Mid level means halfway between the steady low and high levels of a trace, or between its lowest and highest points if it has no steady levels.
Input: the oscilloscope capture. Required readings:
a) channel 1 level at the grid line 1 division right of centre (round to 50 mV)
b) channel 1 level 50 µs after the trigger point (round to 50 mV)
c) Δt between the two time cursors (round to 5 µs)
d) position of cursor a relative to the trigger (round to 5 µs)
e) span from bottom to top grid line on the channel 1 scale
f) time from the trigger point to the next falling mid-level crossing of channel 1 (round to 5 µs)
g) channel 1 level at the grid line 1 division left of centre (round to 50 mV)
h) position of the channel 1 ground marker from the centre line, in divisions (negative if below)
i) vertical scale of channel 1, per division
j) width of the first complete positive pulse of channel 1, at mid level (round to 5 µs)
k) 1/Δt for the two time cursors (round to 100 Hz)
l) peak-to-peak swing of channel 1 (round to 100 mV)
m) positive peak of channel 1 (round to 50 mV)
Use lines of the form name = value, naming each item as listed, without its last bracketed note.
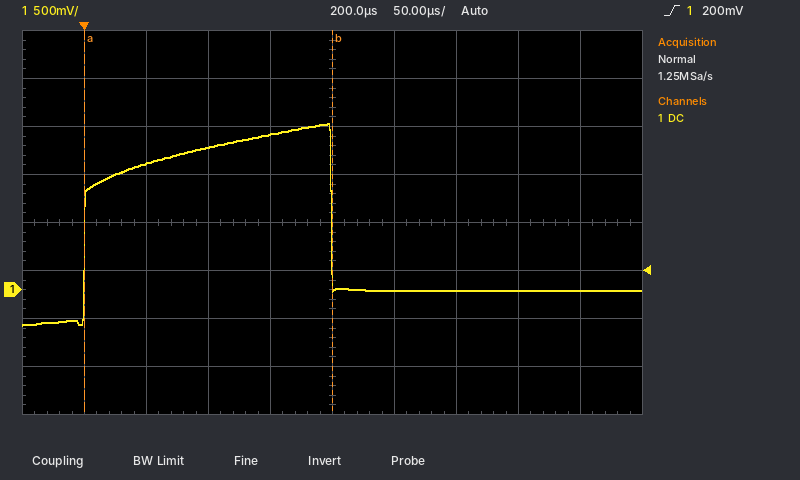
channel 1 level at the grid line 1 division right of centre = 0 mV
channel 1 level 50 µs after the trigger point = 1.30 V
Δt between the two time cursors = 200 µs
position of cursor a relative to the trigger = 0 µs
span from bottom to top grid line on the channel 1 scale = 4 V
time from the trigger point to the next falling mid-level crossing of channel 1 = 200 µs
channel 1 level at the grid line 1 division left of centre = 1.60 V
position of the channel 1 ground marker from the centre line, in divisions = -1.4 div
vertical scale of channel 1, per division = 500 mV
width of the first complete positive pulse of channel 1, at mid level = 200 µs
1/Δt for the two time cursors = 5.0 kHz
peak-to-peak swing of channel 1 = 2.10 V
positive peak of channel 1 = 1.75 V
